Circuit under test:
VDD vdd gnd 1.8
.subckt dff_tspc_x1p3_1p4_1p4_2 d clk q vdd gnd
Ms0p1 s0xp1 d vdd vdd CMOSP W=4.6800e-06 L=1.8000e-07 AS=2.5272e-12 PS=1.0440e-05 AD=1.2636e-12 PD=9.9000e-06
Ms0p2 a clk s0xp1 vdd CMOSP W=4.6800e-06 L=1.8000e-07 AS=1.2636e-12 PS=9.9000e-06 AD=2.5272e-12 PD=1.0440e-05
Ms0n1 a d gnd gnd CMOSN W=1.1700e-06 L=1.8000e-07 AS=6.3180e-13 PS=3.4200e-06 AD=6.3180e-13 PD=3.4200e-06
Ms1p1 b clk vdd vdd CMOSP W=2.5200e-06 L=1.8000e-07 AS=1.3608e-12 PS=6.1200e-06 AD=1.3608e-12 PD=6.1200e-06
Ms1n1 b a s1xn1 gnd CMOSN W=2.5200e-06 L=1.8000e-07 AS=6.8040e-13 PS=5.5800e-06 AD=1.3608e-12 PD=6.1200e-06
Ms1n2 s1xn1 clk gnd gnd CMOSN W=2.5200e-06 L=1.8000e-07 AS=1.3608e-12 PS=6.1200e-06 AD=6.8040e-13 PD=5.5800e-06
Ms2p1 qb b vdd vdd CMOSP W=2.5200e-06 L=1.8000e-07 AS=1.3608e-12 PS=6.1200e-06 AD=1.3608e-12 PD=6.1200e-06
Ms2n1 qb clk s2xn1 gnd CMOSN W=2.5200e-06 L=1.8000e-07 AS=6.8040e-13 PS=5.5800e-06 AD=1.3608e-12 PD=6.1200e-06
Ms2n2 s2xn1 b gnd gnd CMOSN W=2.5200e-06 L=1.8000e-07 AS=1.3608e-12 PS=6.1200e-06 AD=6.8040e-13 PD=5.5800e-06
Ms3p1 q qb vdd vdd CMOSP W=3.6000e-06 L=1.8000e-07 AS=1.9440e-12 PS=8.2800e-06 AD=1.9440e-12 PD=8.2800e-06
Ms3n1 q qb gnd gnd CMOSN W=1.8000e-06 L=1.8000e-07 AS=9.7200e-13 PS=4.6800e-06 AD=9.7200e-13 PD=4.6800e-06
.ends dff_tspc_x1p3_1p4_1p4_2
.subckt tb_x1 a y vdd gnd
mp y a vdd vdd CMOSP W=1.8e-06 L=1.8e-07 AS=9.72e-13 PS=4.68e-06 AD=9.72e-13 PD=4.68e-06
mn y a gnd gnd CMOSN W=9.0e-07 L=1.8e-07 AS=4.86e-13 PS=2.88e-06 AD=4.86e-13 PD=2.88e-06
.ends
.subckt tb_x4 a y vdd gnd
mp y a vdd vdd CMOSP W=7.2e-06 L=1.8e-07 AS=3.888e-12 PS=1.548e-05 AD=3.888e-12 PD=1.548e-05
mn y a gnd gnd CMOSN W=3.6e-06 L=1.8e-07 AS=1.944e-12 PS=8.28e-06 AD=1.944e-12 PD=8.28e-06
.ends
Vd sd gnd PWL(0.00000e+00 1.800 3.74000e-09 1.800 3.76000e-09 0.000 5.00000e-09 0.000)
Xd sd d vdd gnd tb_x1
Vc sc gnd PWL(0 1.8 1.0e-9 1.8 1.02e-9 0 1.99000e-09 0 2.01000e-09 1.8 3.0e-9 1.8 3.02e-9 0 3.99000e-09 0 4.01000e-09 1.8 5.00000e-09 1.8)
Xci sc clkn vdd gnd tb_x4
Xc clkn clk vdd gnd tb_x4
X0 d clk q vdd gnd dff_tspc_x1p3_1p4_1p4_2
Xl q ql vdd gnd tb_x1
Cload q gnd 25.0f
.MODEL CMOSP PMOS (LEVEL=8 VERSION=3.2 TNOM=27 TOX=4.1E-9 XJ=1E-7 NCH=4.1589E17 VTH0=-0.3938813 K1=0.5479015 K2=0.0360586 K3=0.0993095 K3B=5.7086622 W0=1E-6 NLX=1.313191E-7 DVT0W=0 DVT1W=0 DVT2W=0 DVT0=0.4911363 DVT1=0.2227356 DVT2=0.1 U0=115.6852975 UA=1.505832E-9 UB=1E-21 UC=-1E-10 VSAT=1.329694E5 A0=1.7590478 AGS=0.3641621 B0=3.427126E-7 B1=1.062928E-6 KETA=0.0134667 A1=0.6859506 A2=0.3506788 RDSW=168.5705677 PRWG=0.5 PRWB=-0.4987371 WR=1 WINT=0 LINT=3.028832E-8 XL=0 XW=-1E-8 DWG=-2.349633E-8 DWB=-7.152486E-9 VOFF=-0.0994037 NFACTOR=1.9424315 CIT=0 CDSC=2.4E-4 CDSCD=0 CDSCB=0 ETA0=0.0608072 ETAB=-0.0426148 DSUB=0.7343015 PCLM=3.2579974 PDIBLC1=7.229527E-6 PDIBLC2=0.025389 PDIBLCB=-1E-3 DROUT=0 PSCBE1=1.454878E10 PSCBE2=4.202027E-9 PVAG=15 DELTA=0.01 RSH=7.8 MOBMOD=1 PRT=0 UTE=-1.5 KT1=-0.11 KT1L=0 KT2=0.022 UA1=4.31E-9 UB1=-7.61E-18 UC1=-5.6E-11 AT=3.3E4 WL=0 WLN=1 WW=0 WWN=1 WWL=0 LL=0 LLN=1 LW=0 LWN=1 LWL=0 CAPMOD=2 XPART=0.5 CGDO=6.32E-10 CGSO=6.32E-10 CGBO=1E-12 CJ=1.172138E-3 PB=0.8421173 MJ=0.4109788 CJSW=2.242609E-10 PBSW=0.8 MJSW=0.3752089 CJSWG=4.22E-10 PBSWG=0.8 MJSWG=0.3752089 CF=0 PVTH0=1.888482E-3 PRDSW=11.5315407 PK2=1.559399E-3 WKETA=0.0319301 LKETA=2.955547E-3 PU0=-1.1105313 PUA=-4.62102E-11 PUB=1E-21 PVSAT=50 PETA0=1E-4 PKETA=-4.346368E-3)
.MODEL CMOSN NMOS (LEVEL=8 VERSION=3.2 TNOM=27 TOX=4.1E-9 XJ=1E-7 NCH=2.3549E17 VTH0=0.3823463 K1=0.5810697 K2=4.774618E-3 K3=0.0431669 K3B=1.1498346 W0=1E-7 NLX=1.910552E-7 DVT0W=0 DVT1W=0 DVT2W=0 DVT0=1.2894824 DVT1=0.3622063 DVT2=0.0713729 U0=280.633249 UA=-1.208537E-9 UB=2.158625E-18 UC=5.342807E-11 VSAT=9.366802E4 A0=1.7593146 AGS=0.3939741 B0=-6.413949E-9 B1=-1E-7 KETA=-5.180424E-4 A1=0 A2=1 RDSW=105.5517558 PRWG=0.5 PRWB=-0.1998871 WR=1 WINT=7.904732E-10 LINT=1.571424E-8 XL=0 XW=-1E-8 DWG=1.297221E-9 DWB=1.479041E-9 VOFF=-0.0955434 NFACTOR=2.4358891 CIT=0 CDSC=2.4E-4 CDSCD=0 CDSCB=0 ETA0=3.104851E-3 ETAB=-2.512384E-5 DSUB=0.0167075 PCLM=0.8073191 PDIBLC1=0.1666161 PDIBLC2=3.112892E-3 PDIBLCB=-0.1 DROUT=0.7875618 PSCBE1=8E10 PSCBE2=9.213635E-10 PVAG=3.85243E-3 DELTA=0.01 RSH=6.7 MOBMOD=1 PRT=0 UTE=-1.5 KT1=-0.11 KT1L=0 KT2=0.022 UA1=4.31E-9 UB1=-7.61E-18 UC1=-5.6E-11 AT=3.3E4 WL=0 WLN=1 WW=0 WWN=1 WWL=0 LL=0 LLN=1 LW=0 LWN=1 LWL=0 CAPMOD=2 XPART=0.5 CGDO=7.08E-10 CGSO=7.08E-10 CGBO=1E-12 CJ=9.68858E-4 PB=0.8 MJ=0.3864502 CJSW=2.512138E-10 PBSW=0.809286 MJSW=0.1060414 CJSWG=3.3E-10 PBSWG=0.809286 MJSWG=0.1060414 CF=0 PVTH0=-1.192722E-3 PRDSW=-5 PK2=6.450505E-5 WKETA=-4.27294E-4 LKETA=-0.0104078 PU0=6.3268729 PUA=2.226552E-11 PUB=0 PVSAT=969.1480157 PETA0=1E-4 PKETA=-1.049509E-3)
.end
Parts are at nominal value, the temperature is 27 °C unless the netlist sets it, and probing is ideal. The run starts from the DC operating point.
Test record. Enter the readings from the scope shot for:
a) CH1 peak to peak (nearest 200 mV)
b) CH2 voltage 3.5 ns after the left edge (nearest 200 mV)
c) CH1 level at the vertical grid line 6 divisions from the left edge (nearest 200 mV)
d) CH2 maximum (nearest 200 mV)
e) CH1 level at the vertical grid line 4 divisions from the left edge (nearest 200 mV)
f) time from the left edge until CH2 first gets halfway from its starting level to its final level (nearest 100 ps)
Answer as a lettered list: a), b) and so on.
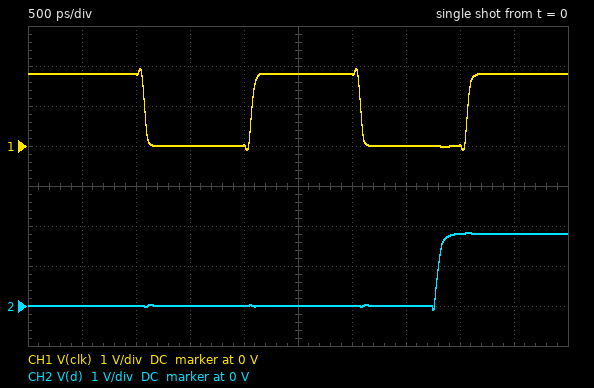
a) 2.0 V
b) 0 V
c) 1.8 V
d) 1.8 V
e) 0 V
f) 3.8 ns
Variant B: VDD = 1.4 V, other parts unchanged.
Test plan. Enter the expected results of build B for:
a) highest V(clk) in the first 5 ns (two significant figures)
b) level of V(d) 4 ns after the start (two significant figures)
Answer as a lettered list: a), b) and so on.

a) 1.5 V
b) 1.4 V
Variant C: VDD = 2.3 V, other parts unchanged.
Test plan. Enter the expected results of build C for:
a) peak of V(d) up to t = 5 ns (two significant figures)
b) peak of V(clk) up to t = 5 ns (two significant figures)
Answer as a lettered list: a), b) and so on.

a) 2.3 V
b) 2.4 V
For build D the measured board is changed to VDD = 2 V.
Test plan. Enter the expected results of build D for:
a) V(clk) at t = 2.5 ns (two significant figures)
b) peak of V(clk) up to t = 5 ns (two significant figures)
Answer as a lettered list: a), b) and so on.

a) 2.0 V
b) 2.1 V
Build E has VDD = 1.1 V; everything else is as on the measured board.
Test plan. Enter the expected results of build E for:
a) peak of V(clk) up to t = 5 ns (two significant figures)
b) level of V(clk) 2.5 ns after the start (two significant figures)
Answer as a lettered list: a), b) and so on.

a) 1.2 V
b) 1.1 V
